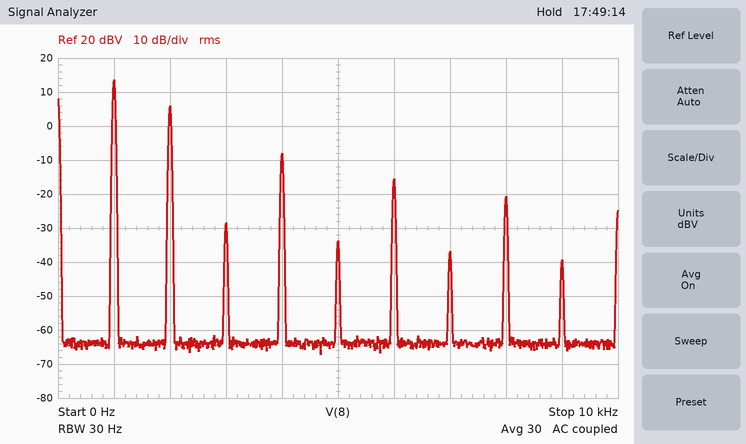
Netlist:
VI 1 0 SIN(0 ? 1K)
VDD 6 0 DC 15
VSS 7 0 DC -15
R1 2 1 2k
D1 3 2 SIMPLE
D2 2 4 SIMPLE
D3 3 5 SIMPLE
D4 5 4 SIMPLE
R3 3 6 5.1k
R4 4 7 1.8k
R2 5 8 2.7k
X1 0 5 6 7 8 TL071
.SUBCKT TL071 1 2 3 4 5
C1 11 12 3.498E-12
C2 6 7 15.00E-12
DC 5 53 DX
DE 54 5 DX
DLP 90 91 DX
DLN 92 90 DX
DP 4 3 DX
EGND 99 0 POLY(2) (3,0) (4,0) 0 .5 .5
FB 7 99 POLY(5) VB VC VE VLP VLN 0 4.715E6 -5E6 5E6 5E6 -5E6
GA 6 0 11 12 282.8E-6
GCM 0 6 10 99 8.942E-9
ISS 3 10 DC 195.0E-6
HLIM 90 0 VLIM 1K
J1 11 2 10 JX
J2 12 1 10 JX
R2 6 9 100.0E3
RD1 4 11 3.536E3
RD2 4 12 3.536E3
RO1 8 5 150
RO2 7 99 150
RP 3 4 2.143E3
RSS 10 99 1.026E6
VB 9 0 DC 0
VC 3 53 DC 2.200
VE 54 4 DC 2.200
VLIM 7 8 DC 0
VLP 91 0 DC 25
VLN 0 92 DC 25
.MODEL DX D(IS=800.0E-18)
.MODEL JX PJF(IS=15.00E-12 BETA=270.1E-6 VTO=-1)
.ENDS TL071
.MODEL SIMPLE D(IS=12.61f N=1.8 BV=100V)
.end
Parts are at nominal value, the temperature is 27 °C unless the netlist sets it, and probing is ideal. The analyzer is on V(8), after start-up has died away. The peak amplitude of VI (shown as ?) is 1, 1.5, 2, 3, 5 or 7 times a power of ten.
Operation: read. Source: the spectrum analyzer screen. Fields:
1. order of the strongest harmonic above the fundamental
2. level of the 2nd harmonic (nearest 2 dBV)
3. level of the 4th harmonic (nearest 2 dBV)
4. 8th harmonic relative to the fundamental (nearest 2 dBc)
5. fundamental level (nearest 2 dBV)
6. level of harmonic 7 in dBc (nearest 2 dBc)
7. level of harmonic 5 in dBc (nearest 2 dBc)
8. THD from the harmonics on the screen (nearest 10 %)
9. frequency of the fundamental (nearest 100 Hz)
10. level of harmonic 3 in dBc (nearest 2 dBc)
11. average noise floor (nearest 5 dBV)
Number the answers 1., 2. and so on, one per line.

1. 2
2. 6 dBV
3. -8 dBV
4. -34 dBc
5. 14 dBV
6. -50 dBc
7. -48 dBc
8. 40 %
9. 1.0 kHz
10. -42 dBc
11. -65 dBV
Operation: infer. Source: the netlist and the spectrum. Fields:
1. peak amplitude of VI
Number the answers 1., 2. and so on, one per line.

1. 10 V
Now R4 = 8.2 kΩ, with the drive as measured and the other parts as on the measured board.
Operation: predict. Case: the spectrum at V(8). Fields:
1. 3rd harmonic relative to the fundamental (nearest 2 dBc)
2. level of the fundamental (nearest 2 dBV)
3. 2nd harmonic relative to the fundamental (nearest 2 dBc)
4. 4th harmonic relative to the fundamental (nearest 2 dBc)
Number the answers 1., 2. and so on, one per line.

1. -12 dBc
2. 14 dBV
3. -20 dBc
4. -26 dBc
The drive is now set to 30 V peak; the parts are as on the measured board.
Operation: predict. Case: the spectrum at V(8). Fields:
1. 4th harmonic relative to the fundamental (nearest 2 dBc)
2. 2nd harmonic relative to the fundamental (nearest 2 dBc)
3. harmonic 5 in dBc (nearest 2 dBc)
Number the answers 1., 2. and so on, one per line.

1. -14 dBc
2. -12 dBc
3. -28 dBc
